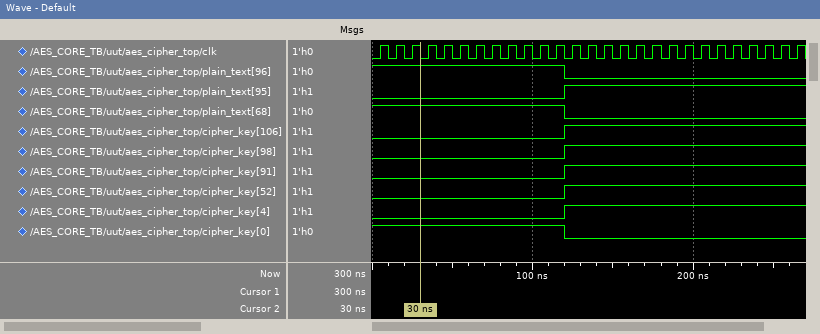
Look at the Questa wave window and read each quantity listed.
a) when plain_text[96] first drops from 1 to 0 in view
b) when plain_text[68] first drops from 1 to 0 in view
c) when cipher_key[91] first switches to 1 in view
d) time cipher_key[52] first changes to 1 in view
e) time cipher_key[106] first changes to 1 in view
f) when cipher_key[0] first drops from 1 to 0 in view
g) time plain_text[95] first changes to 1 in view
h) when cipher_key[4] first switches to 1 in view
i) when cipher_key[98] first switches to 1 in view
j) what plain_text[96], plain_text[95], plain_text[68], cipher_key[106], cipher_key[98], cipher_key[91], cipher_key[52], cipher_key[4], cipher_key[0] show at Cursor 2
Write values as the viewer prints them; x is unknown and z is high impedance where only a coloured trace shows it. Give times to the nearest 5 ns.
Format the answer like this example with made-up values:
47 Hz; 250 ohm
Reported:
120 ns; 120 ns; 120 ns; 120 ns; 120 ns; 120 ns; 120 ns; 120 ns; 120 ns; plain_text[96]=1, plain_text[95]=0, plain_text[68]=1, cipher_key[106]=0, cipher_key[98]=0, cipher_key[91]=0, cipher_key[52]=0, cipher_key[4]=0, cipher_key[0]=1
